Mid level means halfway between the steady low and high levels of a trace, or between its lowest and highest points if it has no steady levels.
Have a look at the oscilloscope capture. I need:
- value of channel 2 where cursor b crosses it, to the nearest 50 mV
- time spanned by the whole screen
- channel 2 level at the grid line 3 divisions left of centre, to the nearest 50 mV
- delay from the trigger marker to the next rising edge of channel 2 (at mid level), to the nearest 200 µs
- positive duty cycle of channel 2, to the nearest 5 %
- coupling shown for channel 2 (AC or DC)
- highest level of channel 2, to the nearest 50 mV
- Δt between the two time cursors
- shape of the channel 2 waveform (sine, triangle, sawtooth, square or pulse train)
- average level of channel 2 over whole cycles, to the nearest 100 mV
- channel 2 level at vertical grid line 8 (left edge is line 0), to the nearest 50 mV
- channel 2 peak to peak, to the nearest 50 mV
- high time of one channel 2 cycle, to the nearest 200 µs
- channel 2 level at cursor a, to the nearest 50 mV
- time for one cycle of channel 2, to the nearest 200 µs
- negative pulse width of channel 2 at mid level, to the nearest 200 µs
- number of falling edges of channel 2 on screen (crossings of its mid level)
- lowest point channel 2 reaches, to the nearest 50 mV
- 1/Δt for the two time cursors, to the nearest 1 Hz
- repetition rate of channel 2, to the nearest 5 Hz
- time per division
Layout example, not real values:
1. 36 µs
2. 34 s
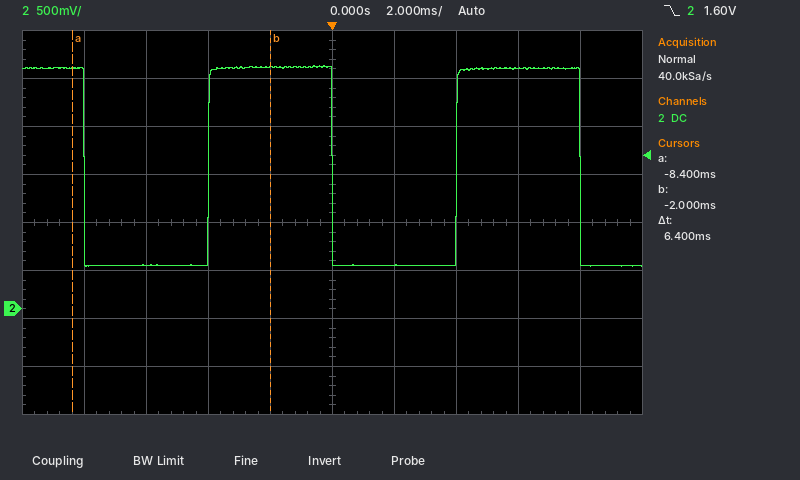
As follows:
1. 2.50 V
2. 20 ms
3. 450 mV
4. 4.0 ms
5. 50 %
6. DC
7. 2.55 V
8. 6.4 ms
9. square
10. 1.5 V
11. 2.50 V
12. 2.10 V
13. 4.0 ms
14. 2.50 V
15. 8.0 ms
16. 4.0 ms
17. 3
18. 450 mV
19. 156 Hz
20. 125 Hz
21. 2 ms
